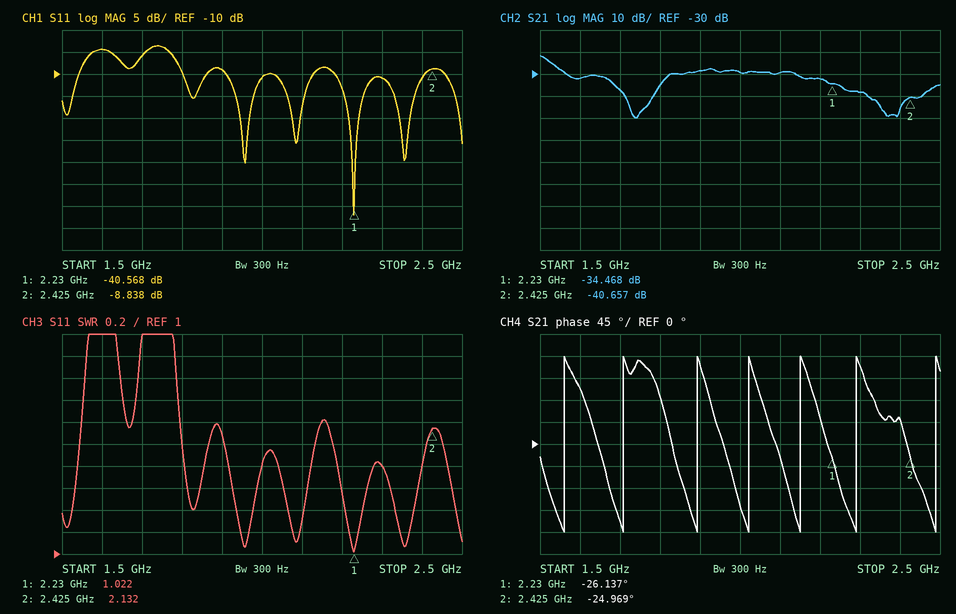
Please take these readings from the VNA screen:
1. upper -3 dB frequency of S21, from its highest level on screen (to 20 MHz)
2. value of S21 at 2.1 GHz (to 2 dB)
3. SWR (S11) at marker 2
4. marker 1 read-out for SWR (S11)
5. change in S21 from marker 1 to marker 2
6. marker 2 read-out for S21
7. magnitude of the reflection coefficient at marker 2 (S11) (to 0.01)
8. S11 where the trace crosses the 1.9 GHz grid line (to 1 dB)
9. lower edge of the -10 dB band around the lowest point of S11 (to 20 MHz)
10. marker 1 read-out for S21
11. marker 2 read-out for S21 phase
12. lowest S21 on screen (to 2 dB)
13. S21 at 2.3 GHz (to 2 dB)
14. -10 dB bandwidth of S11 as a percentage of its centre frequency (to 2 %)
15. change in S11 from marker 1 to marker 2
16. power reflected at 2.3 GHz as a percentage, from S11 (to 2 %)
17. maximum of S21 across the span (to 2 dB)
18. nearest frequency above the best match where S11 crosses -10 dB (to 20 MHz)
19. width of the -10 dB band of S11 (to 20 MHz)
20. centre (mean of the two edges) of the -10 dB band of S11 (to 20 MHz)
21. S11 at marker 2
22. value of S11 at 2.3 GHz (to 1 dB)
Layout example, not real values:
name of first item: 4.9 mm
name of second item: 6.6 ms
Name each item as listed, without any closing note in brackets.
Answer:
upper -3 dB frequency of S21, from its highest level on screen: 1.52 GHz
value of S21 at 2.1 GHz: -30 dB
SWR (S11) at marker 2: 2.132
marker 1 read-out for SWR: 1.022
change in S21 from marker 1 to marker 2: -6.189 dB
marker 2 read-out for S21: -40.657 dB
magnitude of the reflection coefficient at marker 2 (S11): 0.36
S11 where the trace crosses the 1.9 GHz grid line: -9 dB
lower edge of the -10 dB band around the lowest point of S11: 2.18 GHz
marker 1 read-out for S21: -34.468 dB
marker 2 read-out for S21 phase: -24.969°
lowest S21 on screen: -50 dB
S21 at 2.3 GHz: -38 dB
-10 dB bandwidth of S11 as a percentage of its centre frequency: 10 %
change in S11 from marker 1 to marker 2: 31.730 dB
power reflected at 2.3 GHz as a percentage, from S11: 8 %
maximum of S21 across the span: -22 dB
nearest frequency above the best match where S11 crosses -10 dB: 2.40 GHz
width of the -10 dB band of S11: 220 MHz
centre (mean of the two edges) of the -10 dB band of S11: 2.30 GHz
S11 at marker 2: -8.838 dB
value of S11 at 2.3 GHz: -11 dB
